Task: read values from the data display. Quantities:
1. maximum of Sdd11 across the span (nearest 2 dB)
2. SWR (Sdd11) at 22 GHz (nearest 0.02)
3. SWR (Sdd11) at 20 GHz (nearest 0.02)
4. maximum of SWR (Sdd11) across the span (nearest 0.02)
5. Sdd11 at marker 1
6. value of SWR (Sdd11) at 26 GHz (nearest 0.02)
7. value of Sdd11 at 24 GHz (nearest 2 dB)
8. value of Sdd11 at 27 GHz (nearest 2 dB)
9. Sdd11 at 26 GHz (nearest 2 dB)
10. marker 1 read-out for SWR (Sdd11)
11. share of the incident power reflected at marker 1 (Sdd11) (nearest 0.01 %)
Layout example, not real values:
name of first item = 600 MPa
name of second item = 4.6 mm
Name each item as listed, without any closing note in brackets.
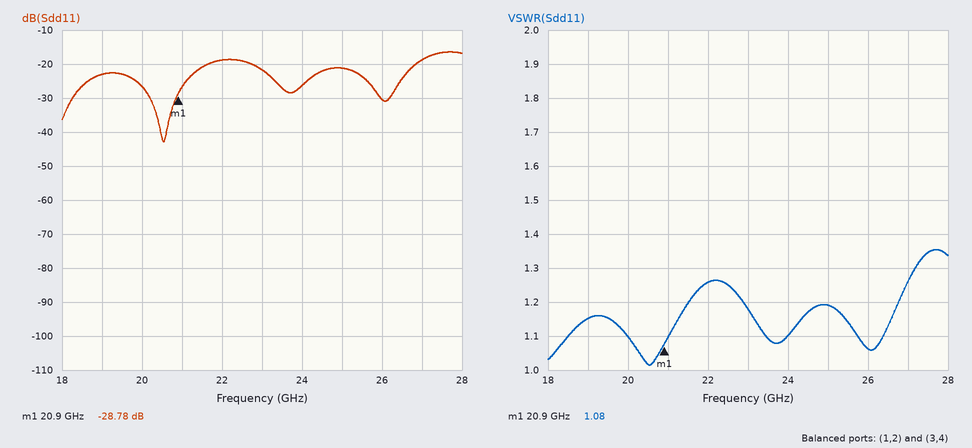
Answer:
maximum of Sdd11 across the span = -16 dB
SWR (Sdd11) at 22 GHz = 1.26
SWR (Sdd11) at 20 GHz = 1.10
maximum of SWR (Sdd11) across the span = 1.36
Sdd11 at marker 1 = -28.78 dB
value of SWR (Sdd11) at 26 GHz = 1.06
value of Sdd11 at 24 GHz = -26 dB
value of Sdd11 at 27 GHz = -18 dB
Sdd11 at 26 GHz = -30 dB
marker 1 read-out for SWR = 1.08
share of the incident power reflected at marker 1 (Sdd11) = 0.13 %
